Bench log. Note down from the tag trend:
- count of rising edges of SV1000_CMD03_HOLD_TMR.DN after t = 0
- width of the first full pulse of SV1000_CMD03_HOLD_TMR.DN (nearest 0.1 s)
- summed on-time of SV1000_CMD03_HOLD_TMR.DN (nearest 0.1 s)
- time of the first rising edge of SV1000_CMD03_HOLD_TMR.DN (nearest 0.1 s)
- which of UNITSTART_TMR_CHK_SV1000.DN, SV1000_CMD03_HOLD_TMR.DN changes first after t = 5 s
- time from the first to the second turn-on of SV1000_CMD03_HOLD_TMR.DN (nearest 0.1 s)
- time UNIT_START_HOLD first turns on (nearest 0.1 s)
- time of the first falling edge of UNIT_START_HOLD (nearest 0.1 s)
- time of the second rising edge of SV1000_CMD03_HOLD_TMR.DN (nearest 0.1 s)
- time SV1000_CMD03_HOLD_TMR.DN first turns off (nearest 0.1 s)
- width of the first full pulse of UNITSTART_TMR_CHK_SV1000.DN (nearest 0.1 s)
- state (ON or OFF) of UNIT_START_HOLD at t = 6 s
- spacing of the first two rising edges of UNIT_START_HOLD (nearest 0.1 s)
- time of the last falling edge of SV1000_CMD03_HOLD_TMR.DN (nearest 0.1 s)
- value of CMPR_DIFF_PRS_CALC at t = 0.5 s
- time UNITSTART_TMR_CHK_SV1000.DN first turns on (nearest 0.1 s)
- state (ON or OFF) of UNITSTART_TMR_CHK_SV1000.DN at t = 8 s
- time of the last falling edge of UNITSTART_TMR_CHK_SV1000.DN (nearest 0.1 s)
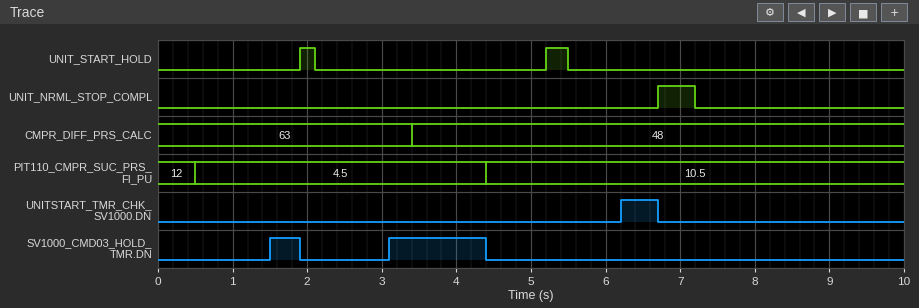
2
0.4 s
1.7 s
1.5 s
UNITSTART_TMR_CHK_SV1000.DN
1.6 s
1.9 s
2.1 s
3.1 s
1.9 s
0.5 s
OFF
3.3 s
4.4 s
63
6.2 s
OFF
6.7 s
